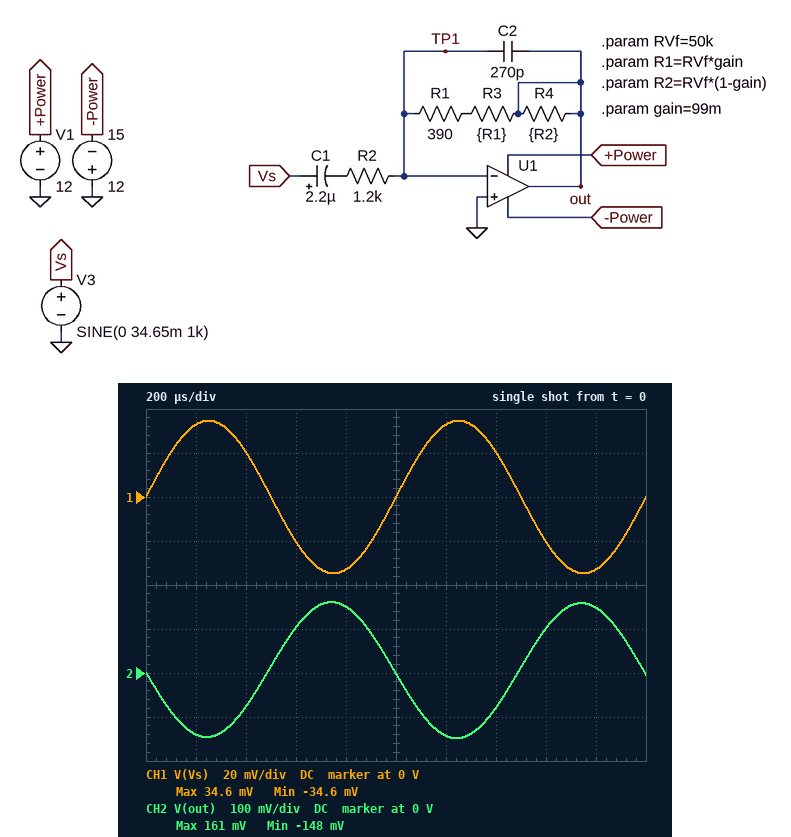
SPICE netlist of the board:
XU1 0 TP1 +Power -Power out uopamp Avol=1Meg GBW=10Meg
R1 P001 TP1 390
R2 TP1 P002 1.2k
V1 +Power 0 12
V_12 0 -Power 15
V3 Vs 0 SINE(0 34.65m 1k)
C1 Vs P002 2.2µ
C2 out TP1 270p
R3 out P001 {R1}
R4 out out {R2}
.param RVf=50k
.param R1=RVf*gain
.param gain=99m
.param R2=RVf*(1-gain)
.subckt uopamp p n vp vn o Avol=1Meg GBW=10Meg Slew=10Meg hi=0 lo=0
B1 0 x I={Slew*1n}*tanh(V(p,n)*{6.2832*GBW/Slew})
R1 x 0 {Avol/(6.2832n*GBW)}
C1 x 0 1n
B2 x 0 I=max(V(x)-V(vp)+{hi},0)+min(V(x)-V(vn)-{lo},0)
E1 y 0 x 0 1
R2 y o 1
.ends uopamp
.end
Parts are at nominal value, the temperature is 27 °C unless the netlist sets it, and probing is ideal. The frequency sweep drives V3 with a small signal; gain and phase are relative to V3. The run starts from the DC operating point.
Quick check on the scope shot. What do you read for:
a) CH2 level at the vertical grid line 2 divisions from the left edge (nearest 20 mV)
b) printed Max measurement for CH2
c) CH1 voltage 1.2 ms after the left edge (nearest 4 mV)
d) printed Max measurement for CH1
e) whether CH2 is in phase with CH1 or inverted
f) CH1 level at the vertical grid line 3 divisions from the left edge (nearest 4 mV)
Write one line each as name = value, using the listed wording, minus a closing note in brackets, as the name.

CH2 level at the vertical grid line 2 divisions from the left edge = -80 mV
printed Max measurement for CH2 = 161 mV
CH1 voltage 1.2 ms after the left edge = 32 mV
printed Max measurement for CH1 = 34.6 mV
whether CH2 is in phase with CH1 or inverted = inverted
CH1 level at the vertical grid line 3 divisions from the left edge = -20 mV
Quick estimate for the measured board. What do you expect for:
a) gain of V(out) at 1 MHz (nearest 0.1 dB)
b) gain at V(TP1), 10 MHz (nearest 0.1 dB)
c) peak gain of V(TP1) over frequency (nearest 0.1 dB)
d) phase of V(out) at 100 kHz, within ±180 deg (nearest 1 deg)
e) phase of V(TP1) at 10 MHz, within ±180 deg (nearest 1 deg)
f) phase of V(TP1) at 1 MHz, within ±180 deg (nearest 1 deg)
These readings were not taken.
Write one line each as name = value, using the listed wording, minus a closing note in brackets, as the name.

gain of V(out) at 1 MHz = -6.7 dB
gain at V(TP1), 10 MHz = -29.4 dB
peak gain of V(TP1) over frequency = -26.7 dB
phase of V(out) at 100 kHz, within ±180 deg = 136 deg
phase of V(TP1) at 10 MHz, within ±180 deg = -42 deg
phase of V(TP1) at 1 MHz, within ±180 deg = 1 deg
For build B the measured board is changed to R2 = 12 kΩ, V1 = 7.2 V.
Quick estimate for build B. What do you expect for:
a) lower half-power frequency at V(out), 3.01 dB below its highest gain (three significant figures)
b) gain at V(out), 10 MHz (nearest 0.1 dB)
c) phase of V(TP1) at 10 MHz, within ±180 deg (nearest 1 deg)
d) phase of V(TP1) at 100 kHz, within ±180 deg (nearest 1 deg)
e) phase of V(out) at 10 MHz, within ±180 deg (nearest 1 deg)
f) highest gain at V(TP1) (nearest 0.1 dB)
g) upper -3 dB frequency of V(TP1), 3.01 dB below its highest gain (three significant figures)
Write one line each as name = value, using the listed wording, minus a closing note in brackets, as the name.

lower half-power frequency at V(out), 3.01 dB below its highest gain = 6.03 Hz
gain at V(out), 10 MHz = -49.1 dB
phase of V(TP1) at 10 MHz, within ±180 deg = -43 deg
phase of V(TP1) at 100 kHz, within ±180 deg = 47 deg
phase of V(out) at 10 MHz, within ±180 deg = 46 deg
highest gain at V(TP1) = -46.3 dB
upper -3 dB frequency of V(TP1), 3.01 dB below its highest gain = 10.3 MHz
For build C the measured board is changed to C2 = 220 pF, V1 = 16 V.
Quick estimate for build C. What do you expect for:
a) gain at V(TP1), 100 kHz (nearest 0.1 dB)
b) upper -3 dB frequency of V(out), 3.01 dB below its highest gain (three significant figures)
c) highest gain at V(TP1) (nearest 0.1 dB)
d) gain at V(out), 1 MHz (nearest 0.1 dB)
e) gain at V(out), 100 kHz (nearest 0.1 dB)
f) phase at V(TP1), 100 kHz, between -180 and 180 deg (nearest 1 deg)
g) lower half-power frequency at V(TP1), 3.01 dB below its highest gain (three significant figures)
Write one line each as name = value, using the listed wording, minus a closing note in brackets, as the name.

gain at V(TP1), 100 kHz = -29.1 dB
upper -3 dB frequency of V(out), 3.01 dB below its highest gain = 128 kHz
highest gain at V(TP1) = -25.0 dB
gain at V(out), 1 MHz = -5.0 dB
gain at V(out), 100 kHz = 10.9 dB
phase at V(TP1), 100 kHz, between -180 and 180 deg = 51 deg
lower half-power frequency at V(TP1), 3.01 dB below its highest gain = 125 kHz
